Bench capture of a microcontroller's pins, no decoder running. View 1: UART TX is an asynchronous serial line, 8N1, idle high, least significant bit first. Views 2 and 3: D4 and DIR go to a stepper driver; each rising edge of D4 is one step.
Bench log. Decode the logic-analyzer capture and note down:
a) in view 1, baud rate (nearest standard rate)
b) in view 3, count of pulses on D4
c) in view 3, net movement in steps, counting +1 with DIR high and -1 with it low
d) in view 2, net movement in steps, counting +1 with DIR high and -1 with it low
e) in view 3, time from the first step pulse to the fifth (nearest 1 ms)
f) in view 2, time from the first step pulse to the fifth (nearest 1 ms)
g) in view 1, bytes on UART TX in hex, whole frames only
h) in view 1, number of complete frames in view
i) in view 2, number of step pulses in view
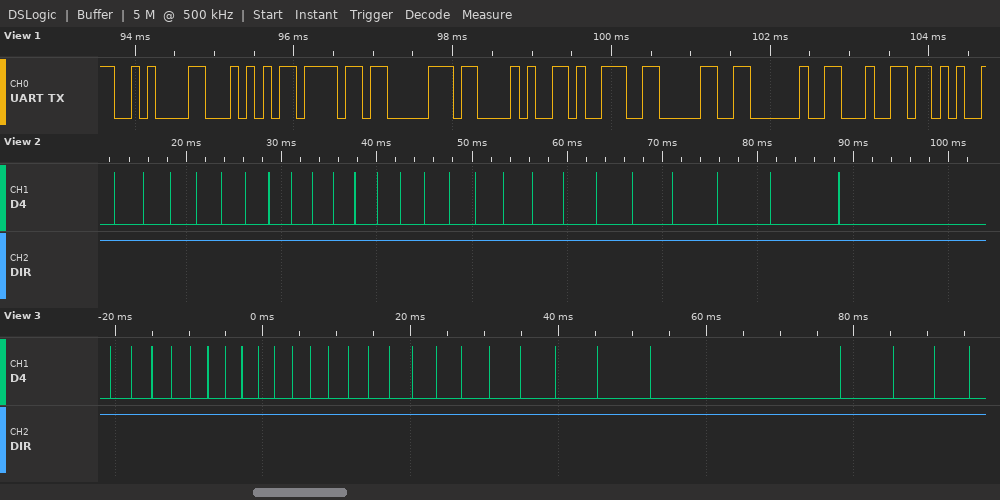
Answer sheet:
9600 baud
28
+28
+25
11 ms
11 ms
0A 54 6F 70 28 39 30 20 64
9
25
